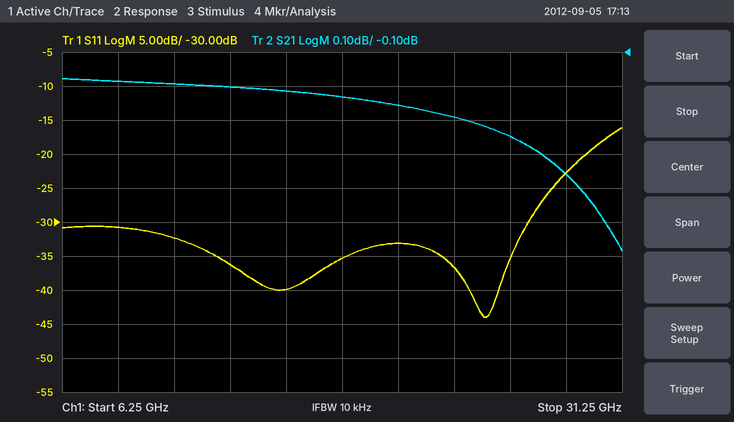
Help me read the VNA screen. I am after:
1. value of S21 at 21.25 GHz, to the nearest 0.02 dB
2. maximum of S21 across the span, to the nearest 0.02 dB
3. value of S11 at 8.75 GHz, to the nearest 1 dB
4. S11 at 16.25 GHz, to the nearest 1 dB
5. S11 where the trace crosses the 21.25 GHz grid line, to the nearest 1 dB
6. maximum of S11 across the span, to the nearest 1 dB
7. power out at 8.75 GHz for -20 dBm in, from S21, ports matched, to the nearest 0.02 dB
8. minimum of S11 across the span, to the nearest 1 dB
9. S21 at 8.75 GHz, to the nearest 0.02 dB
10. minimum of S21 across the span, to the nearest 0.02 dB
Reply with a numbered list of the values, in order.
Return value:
1. -0.26 dB
2. -0.18 dB
3. -31 dB
4. -40 dB
5. -33 dB
6. -16 dB
7. -20.18 dBm
8. -44 dB
9. -0.18 dB
10. -0.68 dB
